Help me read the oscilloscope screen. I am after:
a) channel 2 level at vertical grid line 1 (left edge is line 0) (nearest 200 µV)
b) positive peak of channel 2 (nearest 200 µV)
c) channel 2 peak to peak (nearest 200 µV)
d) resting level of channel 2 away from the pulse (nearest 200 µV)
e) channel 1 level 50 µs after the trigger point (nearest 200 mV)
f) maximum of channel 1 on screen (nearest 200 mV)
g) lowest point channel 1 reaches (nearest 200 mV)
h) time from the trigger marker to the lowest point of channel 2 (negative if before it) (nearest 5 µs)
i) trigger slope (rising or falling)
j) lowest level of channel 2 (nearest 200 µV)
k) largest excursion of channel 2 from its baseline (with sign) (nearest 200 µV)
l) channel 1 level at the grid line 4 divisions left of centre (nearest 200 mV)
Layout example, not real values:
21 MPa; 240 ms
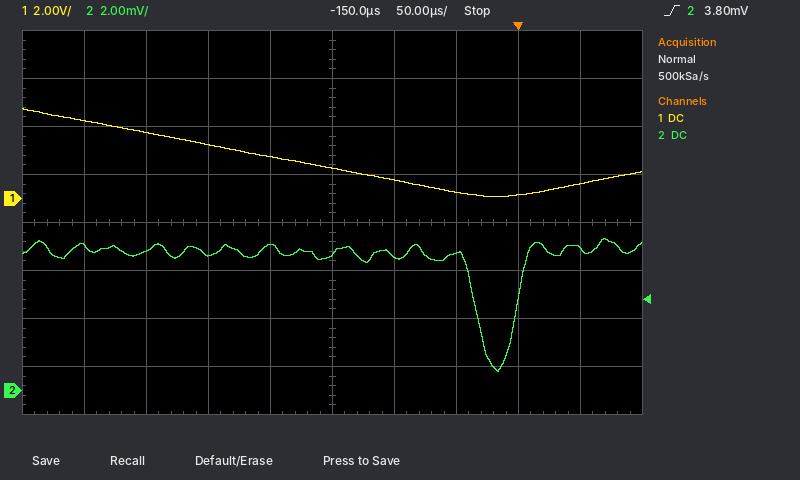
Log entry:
6.0 mV; 6.4 mV; 5.6 mV; 5.8 mV; 600 mV; 3.8 V; 0.0 V; -15 µs; rising; 800 µV; -5.0 mV; 3.2 V
